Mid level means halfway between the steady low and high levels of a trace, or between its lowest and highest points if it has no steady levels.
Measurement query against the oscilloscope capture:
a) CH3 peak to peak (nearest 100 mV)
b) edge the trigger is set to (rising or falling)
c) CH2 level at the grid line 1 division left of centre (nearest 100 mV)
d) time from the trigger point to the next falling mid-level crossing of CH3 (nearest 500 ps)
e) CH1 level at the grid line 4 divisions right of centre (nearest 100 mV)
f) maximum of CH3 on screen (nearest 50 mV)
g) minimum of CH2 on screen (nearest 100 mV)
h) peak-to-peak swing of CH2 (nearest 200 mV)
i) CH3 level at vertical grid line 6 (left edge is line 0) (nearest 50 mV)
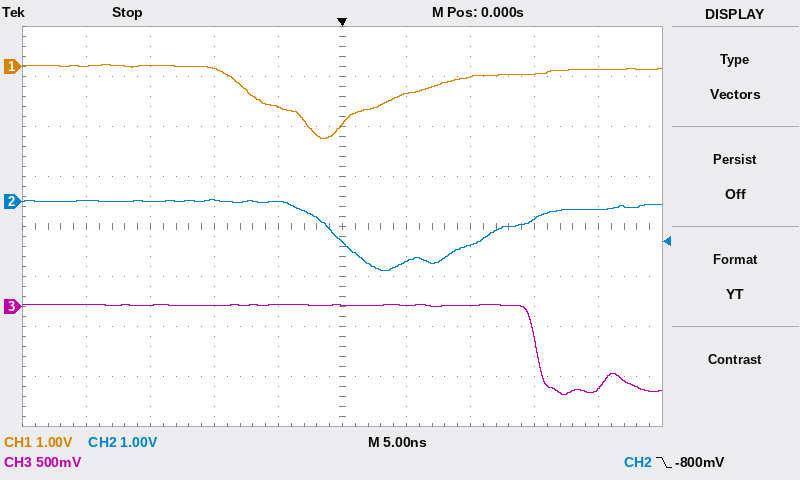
900 mV
falling
0.0 V
15.0 ns
-100 mV
0 mV
-1.4 V
1.4 V
0 mV
